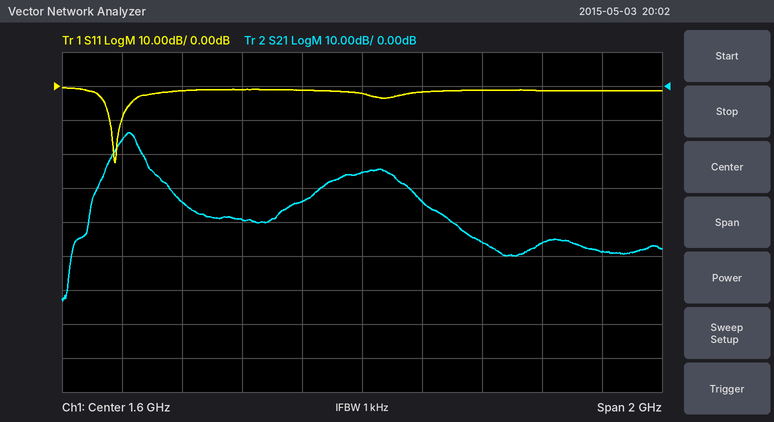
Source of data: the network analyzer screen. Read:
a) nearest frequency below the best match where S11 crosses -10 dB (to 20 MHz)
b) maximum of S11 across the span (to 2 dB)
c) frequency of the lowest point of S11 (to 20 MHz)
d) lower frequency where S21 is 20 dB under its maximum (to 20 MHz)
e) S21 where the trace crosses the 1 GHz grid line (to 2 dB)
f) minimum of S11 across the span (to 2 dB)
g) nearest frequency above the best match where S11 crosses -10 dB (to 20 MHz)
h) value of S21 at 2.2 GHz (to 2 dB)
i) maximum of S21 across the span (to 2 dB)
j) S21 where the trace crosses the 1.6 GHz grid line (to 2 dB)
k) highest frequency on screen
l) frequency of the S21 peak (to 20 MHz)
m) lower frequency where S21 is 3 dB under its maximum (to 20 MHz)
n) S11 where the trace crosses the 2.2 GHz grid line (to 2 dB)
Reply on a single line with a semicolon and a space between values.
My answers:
760 MHz; 0 dB; 780 MHz; 700 MHz; -34 dB; -22 dB; 800 MHz; -46 dB; -14 dB; -26 dB; 2.6 GHz; 820 MHz; 800 MHz; -2 dB
